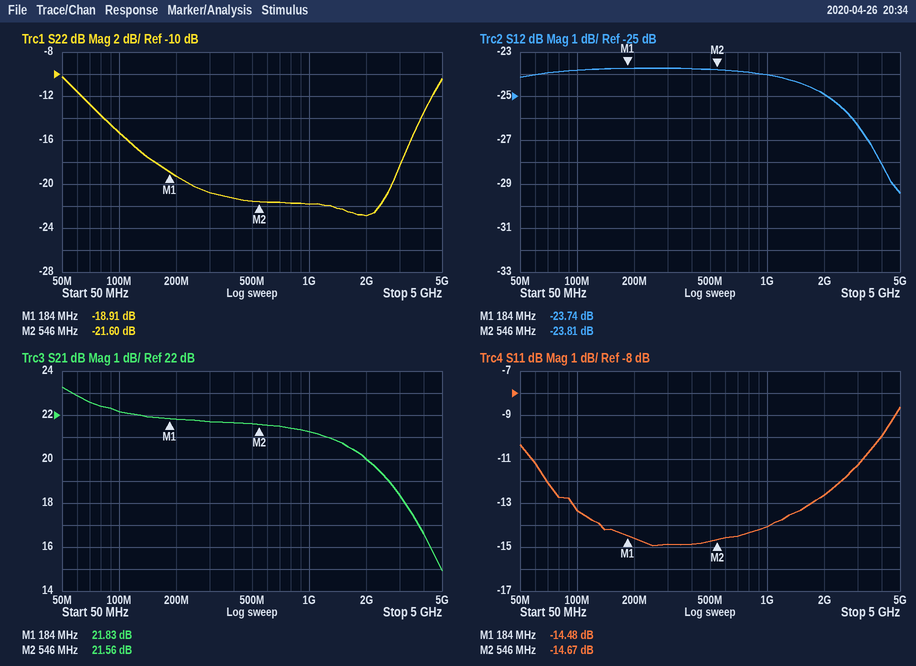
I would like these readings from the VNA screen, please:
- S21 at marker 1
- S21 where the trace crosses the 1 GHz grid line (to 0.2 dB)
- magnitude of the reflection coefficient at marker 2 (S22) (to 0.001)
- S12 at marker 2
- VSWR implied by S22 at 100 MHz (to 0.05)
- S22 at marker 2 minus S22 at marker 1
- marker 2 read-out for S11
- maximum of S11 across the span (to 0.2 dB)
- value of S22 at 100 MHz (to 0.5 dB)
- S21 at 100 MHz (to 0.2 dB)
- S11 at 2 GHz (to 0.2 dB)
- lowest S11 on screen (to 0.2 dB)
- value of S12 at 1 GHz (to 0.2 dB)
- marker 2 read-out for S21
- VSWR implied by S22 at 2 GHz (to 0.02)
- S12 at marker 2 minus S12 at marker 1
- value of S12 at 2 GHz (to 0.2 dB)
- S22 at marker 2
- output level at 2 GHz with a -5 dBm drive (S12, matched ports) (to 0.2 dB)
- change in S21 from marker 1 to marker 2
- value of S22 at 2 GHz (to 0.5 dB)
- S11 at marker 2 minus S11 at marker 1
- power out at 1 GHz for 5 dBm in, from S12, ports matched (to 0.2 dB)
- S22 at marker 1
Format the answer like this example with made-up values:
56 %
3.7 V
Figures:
21.83 dB
21.2 dB
0.083
-23.81 dB
1.40
-2.69 dB
-14.67 dB
-8.6 dB
-15.5 dB
22.2 dB
-12.6 dB
-15.0 dB
-24.0 dB
21.56 dB
1.16
-0.07 dB
-25.0 dB
-21.60 dB
-30.0 dBm
-0.27 dB
-23.0 dB
-0.19 dB
-19.0 dBm
-18.91 dB
